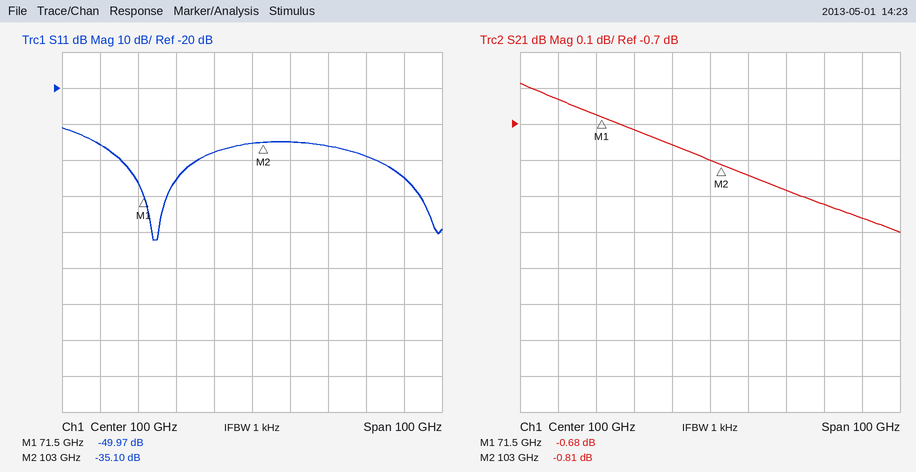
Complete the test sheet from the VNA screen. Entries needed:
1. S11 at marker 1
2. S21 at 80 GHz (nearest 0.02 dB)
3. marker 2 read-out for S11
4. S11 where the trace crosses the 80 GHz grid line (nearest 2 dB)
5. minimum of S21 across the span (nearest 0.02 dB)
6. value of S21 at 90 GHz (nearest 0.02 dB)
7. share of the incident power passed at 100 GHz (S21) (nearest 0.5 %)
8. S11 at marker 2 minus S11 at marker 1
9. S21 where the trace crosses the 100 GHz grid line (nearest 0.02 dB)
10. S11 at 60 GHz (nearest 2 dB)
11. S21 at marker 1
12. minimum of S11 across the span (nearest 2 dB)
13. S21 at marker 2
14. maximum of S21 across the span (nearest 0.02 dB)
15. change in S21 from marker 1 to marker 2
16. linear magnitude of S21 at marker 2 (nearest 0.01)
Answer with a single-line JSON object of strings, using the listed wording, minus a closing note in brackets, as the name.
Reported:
{"S11 at marker 1": "-49.97 dB", "S21 at 80 GHz": "-0.72 dB", "marker 2 read-out for S11": "-35.10 dB", "S11 where the trace crosses the 80 GHz grid line": "-46 dB", "minimum of S21 across the span": "-1.00 dB", "value of S21 at 90 GHz": "-0.76 dB", "share of the incident power passed at 100 GHz (S21)": "83.0 %", "S11 at marker 2 minus S11 at marker 1": "14.87 dB", "S21 where the trace crosses the 100 GHz grid line": "-0.80 dB", "S11 at 60 GHz": "-36 dB", "S21 at marker 1": "-0.68 dB", "minimum of S11 across the span": "-62 dB", "S21 at marker 2": "-0.81 dB", "maximum of S21 across the span": "-0.58 dB", "change in S21 from marker 1 to marker 2": "-0.13 dB", "linear magnitude of S21 at marker 2": "0.91"}
